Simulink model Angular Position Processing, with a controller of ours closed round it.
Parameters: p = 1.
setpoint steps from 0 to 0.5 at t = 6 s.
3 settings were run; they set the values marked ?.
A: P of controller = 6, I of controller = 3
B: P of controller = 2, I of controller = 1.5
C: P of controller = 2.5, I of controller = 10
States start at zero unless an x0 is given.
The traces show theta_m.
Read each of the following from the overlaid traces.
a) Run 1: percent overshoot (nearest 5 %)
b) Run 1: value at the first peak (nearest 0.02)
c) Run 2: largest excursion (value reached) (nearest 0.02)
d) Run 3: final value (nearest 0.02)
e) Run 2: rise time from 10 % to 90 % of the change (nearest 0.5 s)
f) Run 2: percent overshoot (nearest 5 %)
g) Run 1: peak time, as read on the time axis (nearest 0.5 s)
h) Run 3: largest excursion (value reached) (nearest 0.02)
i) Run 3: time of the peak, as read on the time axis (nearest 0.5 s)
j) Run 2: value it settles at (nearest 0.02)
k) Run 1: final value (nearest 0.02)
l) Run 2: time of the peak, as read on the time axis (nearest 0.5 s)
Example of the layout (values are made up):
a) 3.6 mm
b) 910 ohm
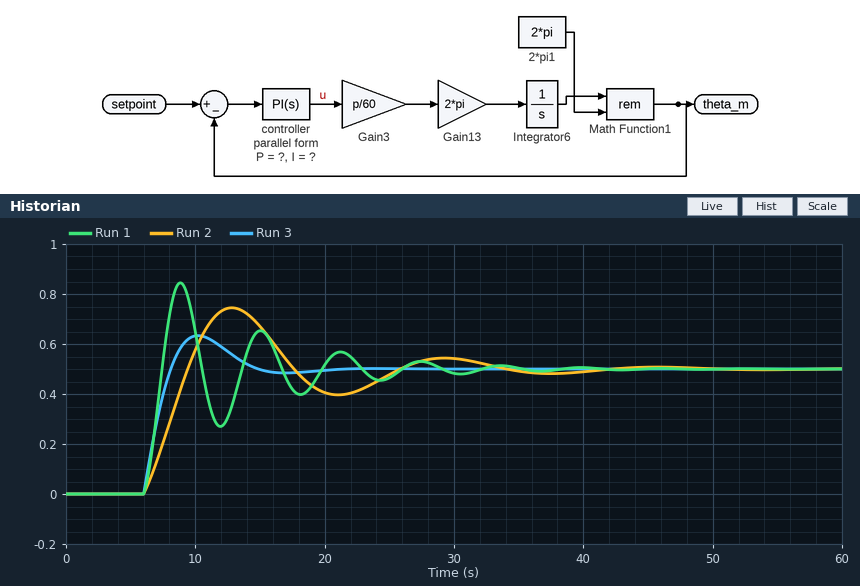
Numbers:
a) 70 %
b) 0.84
c) 0.74
d) 0.50
e) 2.5 s
f) 50 %
g) 9.0 s
h) 0.64
i) 10.0 s
j) 0.50
k) 0.50
l) 13.0 s
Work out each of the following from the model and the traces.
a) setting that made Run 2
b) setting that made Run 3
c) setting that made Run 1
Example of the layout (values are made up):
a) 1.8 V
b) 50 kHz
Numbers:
a) B
b) A
c) C
